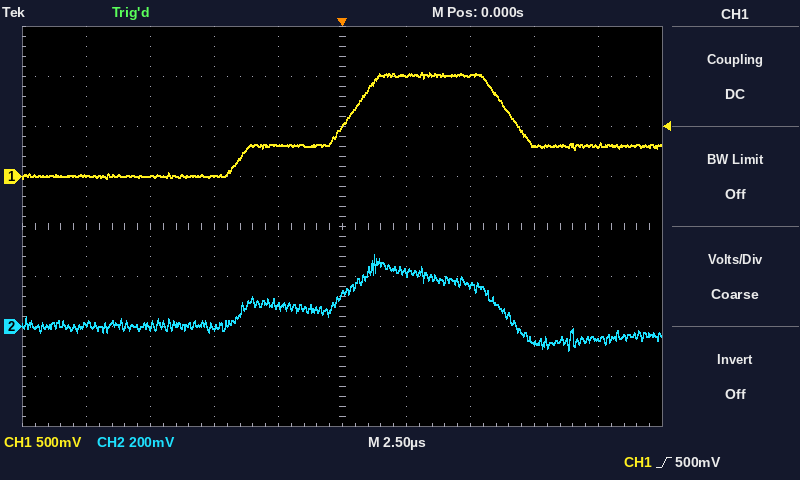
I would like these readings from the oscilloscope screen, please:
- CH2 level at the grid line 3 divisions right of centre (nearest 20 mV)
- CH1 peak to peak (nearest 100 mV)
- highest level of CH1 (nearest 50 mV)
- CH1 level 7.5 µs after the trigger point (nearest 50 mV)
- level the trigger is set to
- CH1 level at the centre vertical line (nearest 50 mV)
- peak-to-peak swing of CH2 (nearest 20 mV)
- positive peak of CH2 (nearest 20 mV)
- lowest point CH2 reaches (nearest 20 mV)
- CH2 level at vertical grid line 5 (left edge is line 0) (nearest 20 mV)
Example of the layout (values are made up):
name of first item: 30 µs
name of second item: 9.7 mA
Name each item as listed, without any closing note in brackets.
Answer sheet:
CH2 level at the grid line 3 divisions right of centre: -60 mV
CH1 peak to peak: 1.10 V
highest level of CH1: 1.05 V
CH1 level 7.5 µs after the trigger point: 300 mV
level the trigger is set to: 500 mV
CH1 level at the centre vertical line: 500 mV
peak-to-peak swing of CH2: 380 mV
positive peak of CH2: 280 mV
lowest point CH2 reaches: -100 mV
CH2 level at vertical grid line 5 (left edge is line 0): 120 mV
